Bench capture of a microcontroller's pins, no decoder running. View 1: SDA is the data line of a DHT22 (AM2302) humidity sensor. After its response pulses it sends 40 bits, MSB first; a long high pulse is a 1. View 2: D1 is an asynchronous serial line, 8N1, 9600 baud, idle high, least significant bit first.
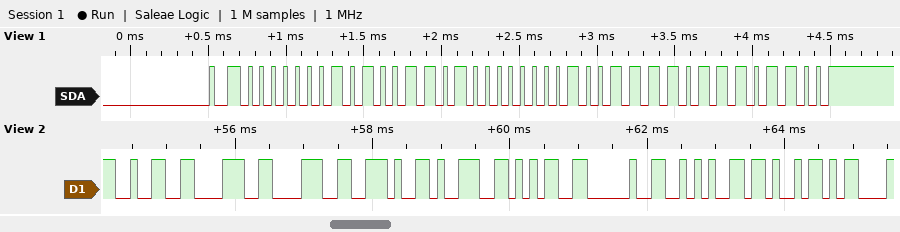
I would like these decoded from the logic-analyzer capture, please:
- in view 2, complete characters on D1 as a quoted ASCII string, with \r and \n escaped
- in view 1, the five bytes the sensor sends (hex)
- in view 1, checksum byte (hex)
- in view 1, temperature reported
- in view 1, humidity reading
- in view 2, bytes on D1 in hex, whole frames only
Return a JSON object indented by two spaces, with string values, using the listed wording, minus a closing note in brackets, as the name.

{
  "in view 2, complete characters on D1 as a quoted ASCII string, with \\r and \\n escaped": "\"288.95 *K\\r\"",
  "in view 1, the five bytes the sensor sends": "01 4D 00 9E EC",
  "in view 1, checksum byte": "0xEC",
  "in view 1, temperature reported": "15.8 °C",
  "in view 1, humidity reading": "33.3 %",
  "in view 2, bytes on D1 in hex, whole frames only": "32 38 38 2E 39 35 20 2A 4B 0D"
}
